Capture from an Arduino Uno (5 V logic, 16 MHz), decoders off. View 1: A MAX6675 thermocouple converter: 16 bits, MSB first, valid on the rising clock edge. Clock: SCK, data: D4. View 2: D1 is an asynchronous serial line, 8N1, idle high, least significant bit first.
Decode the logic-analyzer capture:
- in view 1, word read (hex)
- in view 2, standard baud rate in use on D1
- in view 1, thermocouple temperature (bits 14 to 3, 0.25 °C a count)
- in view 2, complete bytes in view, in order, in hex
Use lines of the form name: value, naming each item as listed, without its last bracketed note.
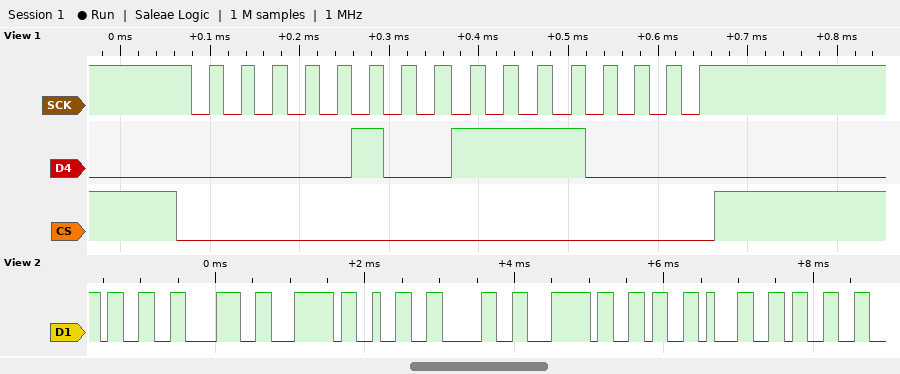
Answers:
in view 1, word read: 0x04F0
in view 2, standard baud rate in use on D1: 9600 baud
in view 1, thermocouple temperature: 39.50 °C
in view 2, complete bytes in view, in order, in hex: 33 38 7C 32 30 7C 36 31 33
